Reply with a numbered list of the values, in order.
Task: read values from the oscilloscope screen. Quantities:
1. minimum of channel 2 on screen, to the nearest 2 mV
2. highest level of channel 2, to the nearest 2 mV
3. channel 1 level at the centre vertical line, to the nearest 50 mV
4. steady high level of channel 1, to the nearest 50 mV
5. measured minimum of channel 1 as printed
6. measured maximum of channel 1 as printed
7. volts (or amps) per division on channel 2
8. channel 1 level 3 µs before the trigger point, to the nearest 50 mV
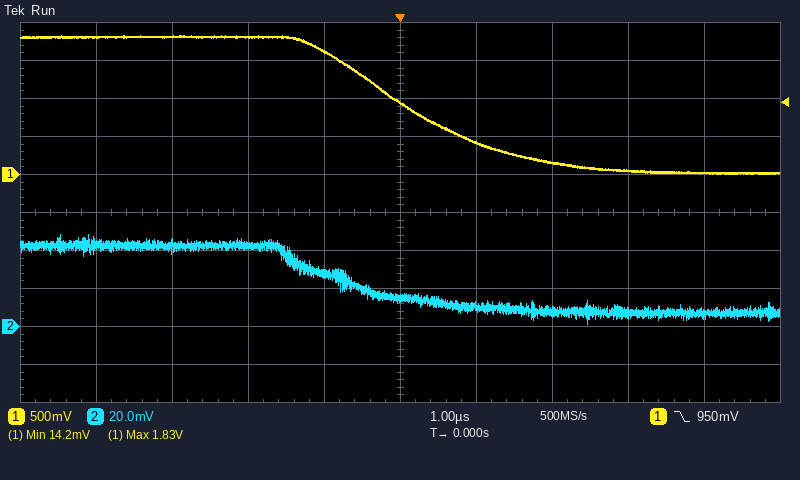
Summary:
1. 2 mV
2. 48 mV
3. 950 mV
4. 1.80 V
5. 14.2 mV
6. 1.83 V
7. 20 mV
8. 1.80 V
